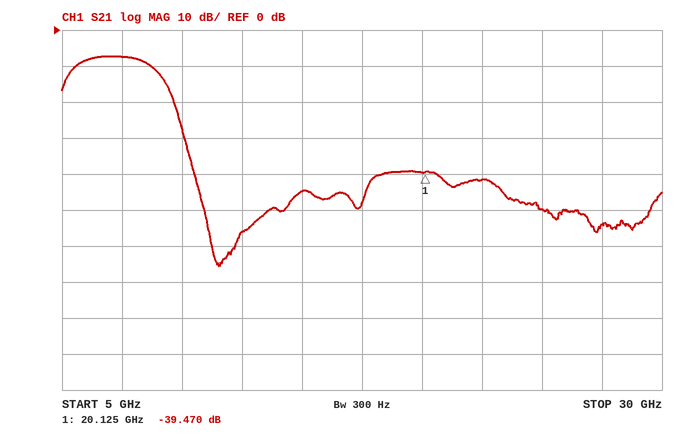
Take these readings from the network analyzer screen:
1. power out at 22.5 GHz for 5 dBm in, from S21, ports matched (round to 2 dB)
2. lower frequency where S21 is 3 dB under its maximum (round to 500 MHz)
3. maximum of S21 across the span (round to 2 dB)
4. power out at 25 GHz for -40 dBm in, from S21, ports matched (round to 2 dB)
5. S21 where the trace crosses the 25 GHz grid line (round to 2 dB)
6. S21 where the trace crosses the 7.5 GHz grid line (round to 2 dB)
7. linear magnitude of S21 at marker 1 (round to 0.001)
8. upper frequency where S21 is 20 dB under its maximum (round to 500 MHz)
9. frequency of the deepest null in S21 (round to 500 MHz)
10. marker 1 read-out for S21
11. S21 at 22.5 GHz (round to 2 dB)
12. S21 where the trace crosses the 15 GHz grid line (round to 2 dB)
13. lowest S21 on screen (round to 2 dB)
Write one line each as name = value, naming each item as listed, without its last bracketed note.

power out at 22.5 GHz for 5 dBm in, from S21, ports matched = -36 dBm
lower frequency where S21 is 3 dB under its maximum = 5.5 GHz
maximum of S21 across the span = -8 dB
power out at 25 GHz for -40 dBm in, from S21, ports matched = -90 dBm
S21 where the trace crosses the 25 GHz grid line = -50 dB
S21 where the trace crosses the 7.5 GHz grid line = -8 dB
linear magnitude of S21 at marker 1 = 0.011
upper frequency where S21 is 20 dB under its maximum = 10.0 GHz
frequency of the deepest null in S21 = 11.5 GHz
marker 1 read-out for S21 = -39.470 dB
S21 at 22.5 GHz = -42 dB
S21 where the trace crosses the 15 GHz grid line = -44 dB
lowest S21 on screen = -66 dB
